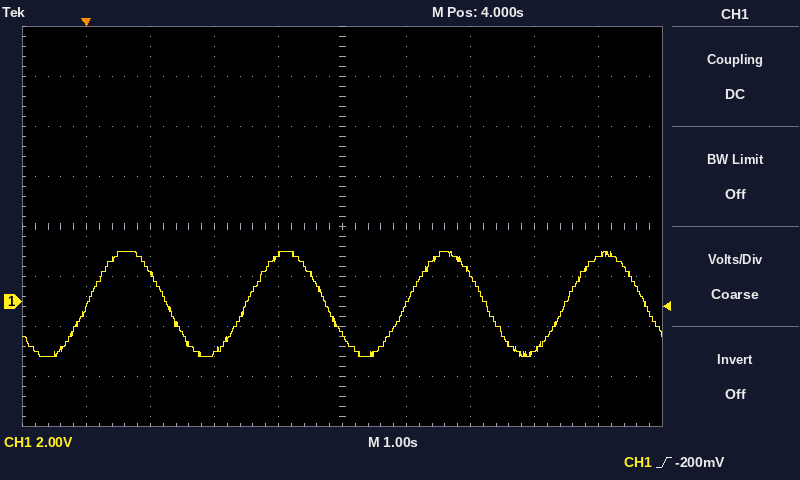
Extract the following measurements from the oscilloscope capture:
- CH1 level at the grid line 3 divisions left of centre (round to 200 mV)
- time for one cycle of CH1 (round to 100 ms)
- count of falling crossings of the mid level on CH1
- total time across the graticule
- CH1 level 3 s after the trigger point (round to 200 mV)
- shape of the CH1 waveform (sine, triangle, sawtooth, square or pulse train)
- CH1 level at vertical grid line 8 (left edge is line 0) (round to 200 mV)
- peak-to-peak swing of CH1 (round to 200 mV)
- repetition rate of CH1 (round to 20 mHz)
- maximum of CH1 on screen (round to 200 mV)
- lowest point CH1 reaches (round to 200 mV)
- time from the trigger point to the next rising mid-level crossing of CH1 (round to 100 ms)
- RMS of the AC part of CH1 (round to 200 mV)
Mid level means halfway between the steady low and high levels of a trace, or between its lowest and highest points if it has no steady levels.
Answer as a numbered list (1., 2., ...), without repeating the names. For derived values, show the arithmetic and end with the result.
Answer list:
1. 1.2 V
2. 2.5 s
3. 4
4. 10 s
5. 1.8 V
6. sine
7. -2.0 V
8. 2.0 V − (-2.2 V) = 4.2 V
9. 1 / 2.5 s ≈ 400 mHz
10. 2.0 V
11. -2.2 V
12. 2.5 s
13. 4.2 V / (2√2) ≈ 1.48 V, so 1.4 V to the nearest 200 mV
